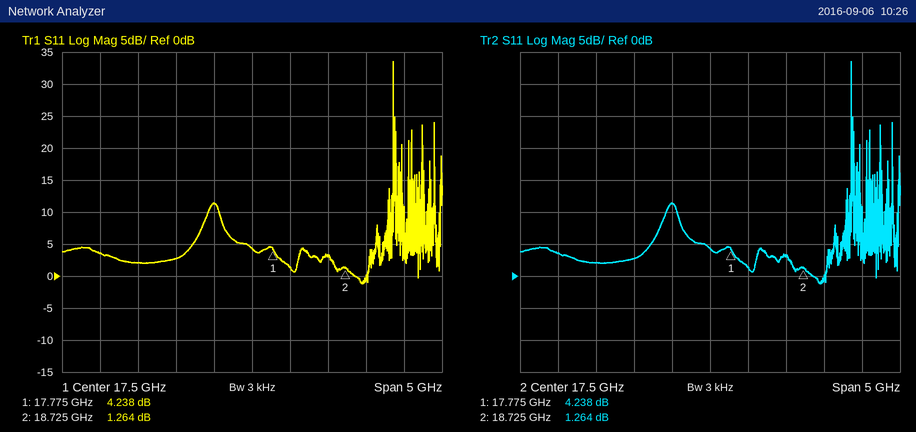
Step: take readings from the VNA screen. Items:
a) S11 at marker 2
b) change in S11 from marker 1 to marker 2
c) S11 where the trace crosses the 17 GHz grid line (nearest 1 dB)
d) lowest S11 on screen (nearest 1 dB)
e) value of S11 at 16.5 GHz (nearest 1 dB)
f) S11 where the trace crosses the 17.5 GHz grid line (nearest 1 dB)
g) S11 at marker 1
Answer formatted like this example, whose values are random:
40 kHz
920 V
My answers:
1.264 dB
-2.974 dB
11 dB
-1 dB
3 dB
4 dB
4.238 dB
